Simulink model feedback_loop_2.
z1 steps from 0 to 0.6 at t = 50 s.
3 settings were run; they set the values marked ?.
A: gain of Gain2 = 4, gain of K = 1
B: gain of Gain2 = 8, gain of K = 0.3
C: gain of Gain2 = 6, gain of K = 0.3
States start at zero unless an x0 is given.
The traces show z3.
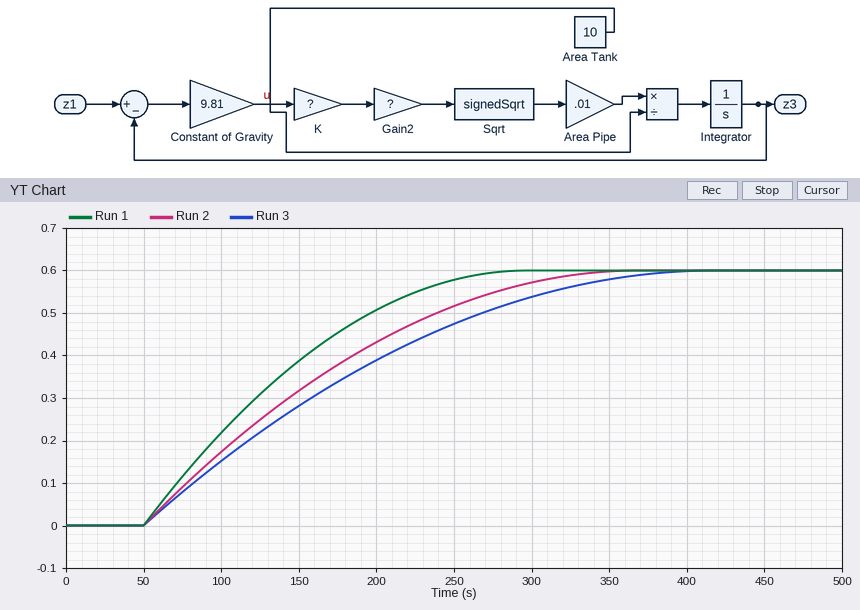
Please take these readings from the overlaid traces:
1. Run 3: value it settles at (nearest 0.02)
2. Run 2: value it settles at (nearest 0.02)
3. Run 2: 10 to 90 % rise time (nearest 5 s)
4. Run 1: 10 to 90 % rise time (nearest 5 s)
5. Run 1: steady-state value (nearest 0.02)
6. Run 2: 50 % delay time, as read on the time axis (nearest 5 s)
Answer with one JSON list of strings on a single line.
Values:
["0.60", "0.60", "200 s", "155 s", "0.60", "145 s"]
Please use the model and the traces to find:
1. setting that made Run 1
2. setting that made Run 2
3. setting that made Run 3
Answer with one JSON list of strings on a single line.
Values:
["A", "B", "C"]
